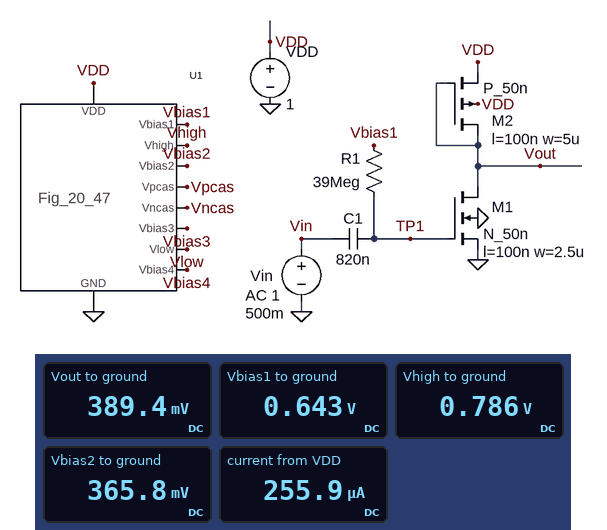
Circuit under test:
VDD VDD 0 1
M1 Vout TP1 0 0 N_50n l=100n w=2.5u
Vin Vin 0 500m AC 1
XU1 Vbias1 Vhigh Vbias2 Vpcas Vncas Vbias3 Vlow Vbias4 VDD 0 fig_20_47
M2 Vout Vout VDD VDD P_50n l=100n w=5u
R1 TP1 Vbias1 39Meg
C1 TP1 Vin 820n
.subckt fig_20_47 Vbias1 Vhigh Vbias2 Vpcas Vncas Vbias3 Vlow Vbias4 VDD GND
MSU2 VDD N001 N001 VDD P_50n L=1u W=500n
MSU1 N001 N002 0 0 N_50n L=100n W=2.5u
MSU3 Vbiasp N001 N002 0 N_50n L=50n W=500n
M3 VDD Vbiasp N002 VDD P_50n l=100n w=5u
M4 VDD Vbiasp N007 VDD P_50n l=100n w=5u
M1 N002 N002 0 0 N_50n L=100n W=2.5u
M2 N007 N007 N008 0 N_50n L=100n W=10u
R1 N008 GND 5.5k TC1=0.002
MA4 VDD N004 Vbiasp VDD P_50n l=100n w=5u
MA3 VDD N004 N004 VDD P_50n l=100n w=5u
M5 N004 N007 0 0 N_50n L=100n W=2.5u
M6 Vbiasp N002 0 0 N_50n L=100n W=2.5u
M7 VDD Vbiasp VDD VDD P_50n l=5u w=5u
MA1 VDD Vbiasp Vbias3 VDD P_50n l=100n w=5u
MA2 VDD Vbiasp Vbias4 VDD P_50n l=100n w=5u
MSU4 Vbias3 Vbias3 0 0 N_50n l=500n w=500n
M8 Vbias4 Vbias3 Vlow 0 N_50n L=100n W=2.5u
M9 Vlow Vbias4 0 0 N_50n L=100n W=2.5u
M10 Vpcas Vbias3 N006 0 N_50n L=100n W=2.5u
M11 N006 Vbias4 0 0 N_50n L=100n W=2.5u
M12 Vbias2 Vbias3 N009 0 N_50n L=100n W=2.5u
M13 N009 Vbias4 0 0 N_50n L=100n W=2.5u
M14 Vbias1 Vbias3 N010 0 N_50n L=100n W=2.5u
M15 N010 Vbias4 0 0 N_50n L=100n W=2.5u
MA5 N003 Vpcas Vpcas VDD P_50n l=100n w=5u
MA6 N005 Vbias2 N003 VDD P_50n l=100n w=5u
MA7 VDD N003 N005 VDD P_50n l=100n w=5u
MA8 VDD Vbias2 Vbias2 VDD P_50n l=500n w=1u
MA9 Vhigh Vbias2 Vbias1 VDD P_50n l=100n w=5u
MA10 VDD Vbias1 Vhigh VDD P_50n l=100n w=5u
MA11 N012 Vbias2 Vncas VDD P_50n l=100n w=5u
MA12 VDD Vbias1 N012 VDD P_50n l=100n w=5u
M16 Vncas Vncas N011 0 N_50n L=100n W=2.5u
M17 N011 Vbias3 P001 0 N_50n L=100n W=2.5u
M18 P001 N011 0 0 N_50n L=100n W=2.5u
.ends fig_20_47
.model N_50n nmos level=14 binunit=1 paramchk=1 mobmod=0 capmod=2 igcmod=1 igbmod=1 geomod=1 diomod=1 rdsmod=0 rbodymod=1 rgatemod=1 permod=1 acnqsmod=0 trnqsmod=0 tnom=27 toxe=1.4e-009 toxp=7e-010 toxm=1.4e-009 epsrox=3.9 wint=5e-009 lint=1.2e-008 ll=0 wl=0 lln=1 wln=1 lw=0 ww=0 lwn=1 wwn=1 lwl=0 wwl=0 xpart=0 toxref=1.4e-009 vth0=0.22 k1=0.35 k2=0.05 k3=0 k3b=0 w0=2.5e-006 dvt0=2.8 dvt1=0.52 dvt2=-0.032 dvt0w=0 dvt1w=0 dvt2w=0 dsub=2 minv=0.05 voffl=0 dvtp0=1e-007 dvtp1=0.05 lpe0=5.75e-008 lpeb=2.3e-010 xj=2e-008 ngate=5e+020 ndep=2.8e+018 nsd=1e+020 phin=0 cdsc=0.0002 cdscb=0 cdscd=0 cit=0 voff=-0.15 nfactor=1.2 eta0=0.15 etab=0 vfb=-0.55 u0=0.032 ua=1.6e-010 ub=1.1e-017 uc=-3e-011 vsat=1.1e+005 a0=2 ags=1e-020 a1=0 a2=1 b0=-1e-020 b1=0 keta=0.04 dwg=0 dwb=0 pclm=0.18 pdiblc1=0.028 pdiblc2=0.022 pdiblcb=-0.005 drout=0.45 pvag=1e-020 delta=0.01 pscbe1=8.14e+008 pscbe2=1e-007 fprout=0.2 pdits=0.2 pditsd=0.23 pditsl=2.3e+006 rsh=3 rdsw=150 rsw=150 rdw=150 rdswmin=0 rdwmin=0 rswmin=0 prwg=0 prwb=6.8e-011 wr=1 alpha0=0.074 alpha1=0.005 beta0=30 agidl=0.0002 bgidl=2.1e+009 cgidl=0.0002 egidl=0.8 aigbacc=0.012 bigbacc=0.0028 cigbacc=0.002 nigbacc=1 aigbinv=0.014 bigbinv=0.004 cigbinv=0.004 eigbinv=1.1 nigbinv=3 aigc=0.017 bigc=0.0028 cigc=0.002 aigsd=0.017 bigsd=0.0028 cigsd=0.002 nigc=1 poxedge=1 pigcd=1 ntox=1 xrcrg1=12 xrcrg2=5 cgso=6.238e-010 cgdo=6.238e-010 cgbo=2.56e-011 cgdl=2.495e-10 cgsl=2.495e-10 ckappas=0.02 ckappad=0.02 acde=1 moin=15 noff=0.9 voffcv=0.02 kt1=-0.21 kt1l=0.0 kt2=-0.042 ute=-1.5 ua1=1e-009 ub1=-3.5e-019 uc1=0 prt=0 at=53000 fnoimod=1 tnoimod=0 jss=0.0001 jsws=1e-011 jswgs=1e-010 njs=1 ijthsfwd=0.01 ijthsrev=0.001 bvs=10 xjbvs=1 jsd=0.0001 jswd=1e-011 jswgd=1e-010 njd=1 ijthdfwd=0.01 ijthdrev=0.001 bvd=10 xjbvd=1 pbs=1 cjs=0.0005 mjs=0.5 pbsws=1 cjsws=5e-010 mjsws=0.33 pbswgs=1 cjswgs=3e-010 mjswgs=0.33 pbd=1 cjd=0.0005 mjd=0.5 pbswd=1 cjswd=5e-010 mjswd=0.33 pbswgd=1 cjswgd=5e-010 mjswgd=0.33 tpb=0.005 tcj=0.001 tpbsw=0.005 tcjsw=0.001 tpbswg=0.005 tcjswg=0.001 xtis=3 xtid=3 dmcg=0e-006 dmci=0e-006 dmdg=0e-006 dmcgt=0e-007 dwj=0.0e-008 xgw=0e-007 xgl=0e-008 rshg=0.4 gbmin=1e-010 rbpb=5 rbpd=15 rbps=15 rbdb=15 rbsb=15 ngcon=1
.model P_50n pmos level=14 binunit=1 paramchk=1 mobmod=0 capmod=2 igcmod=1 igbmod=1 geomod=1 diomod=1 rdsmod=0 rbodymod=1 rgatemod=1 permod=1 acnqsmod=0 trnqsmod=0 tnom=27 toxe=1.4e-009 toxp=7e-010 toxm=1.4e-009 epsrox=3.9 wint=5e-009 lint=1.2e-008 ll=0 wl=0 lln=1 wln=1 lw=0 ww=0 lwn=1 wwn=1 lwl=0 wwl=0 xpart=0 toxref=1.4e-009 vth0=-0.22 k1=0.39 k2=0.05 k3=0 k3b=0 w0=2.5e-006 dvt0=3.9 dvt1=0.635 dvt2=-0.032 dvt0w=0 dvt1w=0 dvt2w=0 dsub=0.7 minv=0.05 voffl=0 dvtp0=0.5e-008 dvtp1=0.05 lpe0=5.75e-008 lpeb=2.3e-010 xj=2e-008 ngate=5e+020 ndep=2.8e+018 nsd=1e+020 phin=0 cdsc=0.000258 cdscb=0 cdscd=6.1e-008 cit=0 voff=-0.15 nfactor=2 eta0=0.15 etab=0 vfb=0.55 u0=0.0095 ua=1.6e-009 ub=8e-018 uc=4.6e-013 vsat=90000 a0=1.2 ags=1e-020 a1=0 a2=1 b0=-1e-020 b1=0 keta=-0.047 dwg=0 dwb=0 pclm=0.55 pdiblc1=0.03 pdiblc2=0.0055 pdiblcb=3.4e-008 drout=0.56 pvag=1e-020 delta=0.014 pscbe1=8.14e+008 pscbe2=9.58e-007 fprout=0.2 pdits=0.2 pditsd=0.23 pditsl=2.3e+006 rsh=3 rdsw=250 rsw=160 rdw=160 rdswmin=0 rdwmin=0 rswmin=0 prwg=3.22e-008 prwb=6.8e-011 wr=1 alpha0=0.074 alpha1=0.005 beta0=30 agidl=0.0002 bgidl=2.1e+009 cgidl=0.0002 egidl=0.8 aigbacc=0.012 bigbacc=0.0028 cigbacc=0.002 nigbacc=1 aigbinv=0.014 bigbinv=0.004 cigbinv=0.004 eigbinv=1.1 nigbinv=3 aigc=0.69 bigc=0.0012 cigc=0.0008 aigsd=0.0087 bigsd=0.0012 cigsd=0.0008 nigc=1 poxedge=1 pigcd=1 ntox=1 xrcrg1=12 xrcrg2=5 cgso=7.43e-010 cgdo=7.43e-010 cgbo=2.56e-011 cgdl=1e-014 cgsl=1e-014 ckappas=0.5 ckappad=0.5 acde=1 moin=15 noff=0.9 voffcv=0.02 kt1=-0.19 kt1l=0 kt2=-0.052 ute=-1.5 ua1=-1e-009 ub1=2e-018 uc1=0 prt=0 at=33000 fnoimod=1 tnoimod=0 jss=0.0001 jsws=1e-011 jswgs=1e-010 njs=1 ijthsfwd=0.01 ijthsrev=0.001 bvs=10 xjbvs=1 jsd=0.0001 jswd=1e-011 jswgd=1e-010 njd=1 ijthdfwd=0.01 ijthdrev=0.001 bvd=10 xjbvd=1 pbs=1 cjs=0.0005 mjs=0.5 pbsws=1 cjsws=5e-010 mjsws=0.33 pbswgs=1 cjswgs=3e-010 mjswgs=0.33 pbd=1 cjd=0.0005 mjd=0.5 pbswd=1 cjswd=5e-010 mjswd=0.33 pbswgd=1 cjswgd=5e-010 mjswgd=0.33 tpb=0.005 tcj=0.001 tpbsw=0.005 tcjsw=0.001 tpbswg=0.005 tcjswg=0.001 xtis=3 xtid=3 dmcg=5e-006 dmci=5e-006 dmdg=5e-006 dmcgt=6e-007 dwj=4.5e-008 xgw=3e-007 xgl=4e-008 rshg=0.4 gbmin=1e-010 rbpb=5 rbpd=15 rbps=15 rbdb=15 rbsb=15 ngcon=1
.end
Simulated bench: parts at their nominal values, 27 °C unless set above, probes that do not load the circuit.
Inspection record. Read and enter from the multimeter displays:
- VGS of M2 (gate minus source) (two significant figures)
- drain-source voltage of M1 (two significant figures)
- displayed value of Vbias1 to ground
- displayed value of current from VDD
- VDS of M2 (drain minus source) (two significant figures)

-610 mV
390 mV
0.643 V
255.9 µA
-610 mV
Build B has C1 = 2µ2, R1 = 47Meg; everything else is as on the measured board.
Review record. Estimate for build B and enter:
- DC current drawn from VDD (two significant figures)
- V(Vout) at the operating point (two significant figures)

250 µA
400 mV
